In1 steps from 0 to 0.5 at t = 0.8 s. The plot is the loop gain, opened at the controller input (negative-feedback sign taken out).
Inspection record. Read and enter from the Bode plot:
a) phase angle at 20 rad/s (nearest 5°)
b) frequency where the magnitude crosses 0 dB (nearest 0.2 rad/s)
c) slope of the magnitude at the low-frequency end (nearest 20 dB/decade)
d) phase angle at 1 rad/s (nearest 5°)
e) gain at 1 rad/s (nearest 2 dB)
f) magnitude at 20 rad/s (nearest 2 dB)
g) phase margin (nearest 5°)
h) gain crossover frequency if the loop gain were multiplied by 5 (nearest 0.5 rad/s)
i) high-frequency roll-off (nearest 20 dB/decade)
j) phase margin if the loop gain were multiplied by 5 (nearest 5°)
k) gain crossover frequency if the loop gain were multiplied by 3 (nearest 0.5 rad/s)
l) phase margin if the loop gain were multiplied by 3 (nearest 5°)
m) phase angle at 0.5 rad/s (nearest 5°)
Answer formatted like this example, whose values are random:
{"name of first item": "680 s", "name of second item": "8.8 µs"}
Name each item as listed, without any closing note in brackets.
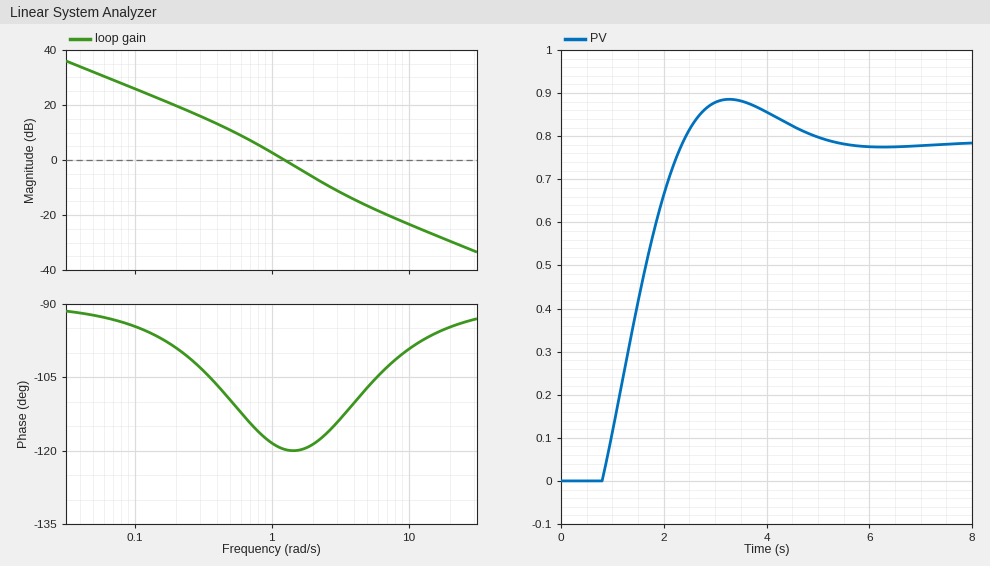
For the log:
{"phase angle at 20 rad/s": "-95°", "frequency where the magnitude crosses 0 dB": "1.2 rad/s", "slope of the magnitude at the low-frequency end": "-20 dB/decade", "phase angle at 1 rad/s": "-120°", "gain at 1 rad/s": "2 dB", "magnitude at 20 rad/s": "-30 dB", "phase margin": "60°", "gain crossover frequency if the loop gain were multiplied by 5": "4.0 rad/s", "high-frequency roll-off": "-20 dB/decade", "phase margin if the loop gain were multiplied by 5": "70°", "gain crossover frequency if the loop gain were multiplied by 3": "2.5 rad/s", "phase margin if the loop gain were multiplied by 3": "65°", "phase angle at 0.5 rad/s": "-110°"}
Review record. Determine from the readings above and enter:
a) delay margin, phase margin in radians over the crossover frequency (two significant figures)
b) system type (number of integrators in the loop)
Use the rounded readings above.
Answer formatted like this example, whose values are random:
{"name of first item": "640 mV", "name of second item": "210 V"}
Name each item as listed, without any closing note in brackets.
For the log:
{"delay margin, phase margin in radians over the crossover frequency": "0.87 s", "system type": "1"}
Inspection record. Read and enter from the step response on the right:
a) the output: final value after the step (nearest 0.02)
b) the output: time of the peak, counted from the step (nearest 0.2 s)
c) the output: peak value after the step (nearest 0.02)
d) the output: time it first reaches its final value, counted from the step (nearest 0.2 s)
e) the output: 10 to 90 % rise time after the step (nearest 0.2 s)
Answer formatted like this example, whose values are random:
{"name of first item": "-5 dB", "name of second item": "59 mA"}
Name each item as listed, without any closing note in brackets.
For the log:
{"the output: final value after the step": "0.78", "the output: time of the peak, counted from the step": "2.4 s", "the output: peak value after the step": "0.88", "the output: time it first reaches its final value, counted from the step": "1.6 s", "the output: 10 to 90 % rise time after the step": "1.2 s"}
